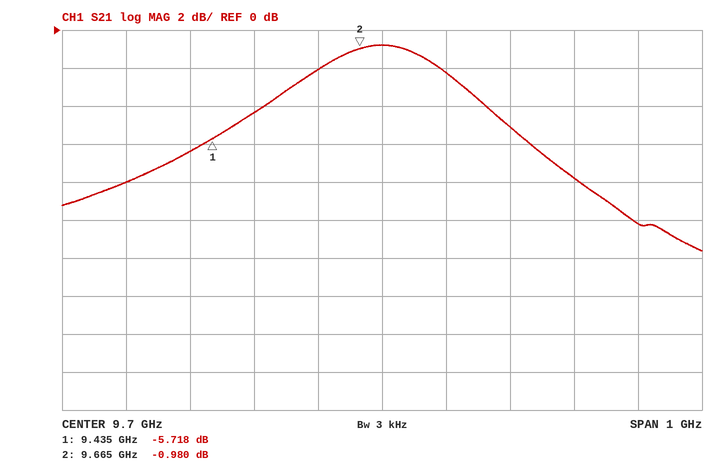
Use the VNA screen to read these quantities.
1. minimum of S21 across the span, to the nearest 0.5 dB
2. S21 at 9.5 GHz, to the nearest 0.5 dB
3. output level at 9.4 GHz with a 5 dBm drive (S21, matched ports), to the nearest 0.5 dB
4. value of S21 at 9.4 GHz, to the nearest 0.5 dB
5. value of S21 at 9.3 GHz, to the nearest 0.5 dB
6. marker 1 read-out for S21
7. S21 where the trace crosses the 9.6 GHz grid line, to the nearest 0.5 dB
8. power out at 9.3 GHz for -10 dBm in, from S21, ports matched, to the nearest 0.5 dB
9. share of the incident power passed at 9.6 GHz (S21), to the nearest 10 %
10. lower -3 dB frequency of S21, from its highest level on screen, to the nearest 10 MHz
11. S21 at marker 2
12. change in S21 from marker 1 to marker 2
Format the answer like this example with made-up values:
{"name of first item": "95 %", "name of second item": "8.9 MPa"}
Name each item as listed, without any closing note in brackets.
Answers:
{"minimum of S21 across the span, to the nearest 0.5 dB": "-11.5 dB", "S21 at 9.5 GHz, to the nearest 0.5 dB": "-4.5 dB", "output level at 9.4 GHz with a 5 dBm drive (S21, matched ports), to the nearest 0.5 dB": "-1.5 dBm", "value of S21 at 9.4 GHz, to the nearest 0.5 dB": "-6.5 dB", "value of S21 at 9.3 GHz, to the nearest 0.5 dB": "-8.0 dB", "marker 1 read-out for S21": "-5.718 dB", "S21 where the trace crosses the 9.6 GHz grid line, to the nearest 0.5 dB": "-2.0 dB", "power out at 9.3 GHz for -10 dBm in, from S21, ports matched, to the nearest 0.5 dB": "-18.0 dBm", "share of the incident power passed at 9.6 GHz (S21), to the nearest 10 %": "60 %", "lower -3 dB frequency of S21, from its highest level on screen, to the nearest 10 MHz": "9.53 GHz", "S21 at marker 2": "-0.980 dB", "change in S21 from marker 1 to marker 2": "4.738 dB"}
